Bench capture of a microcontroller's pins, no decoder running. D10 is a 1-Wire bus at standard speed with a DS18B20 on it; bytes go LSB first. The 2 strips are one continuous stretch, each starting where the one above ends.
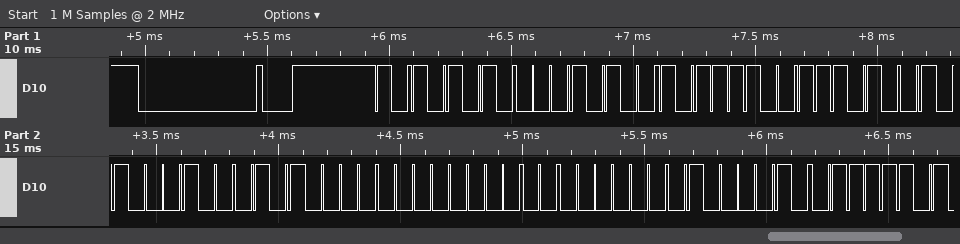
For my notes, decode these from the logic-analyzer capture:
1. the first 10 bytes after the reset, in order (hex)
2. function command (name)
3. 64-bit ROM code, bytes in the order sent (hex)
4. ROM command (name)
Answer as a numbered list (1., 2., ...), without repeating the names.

1. 55 28 3D 97 22 0A 00 00 42 BE
2. Read Scratchpad
3. 28 3D 97 22 0A 00 00 42
4. Match ROM
